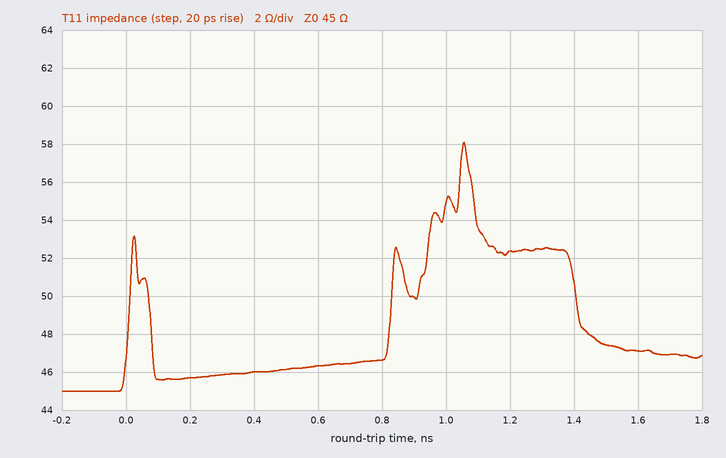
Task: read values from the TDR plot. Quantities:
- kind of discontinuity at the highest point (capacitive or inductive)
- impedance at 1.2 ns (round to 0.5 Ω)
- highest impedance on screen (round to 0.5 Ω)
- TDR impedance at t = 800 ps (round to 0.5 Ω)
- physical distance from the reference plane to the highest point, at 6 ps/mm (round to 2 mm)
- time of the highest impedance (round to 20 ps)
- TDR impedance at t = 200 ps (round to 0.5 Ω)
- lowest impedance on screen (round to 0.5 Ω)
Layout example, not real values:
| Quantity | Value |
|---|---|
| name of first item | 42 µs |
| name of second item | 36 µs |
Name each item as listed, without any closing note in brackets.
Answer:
| Quantity | Value |
|---|---|
| kind of discontinuity at the highest point | inductive |
| impedance at 1.2 ns | 52.5 Ω |
| highest impedance on screen | 58.0 Ω |
| TDR impedance at t = 800 ps | 46.5 Ω |
| physical distance from the reference plane to the highest point, at 6 ps/mm | 88 mm |
| time of the highest impedance | 1.06 ns |
| TDR impedance at t = 200 ps | 45.5 Ω |
| lowest impedance on screen | 45.0 Ω |
